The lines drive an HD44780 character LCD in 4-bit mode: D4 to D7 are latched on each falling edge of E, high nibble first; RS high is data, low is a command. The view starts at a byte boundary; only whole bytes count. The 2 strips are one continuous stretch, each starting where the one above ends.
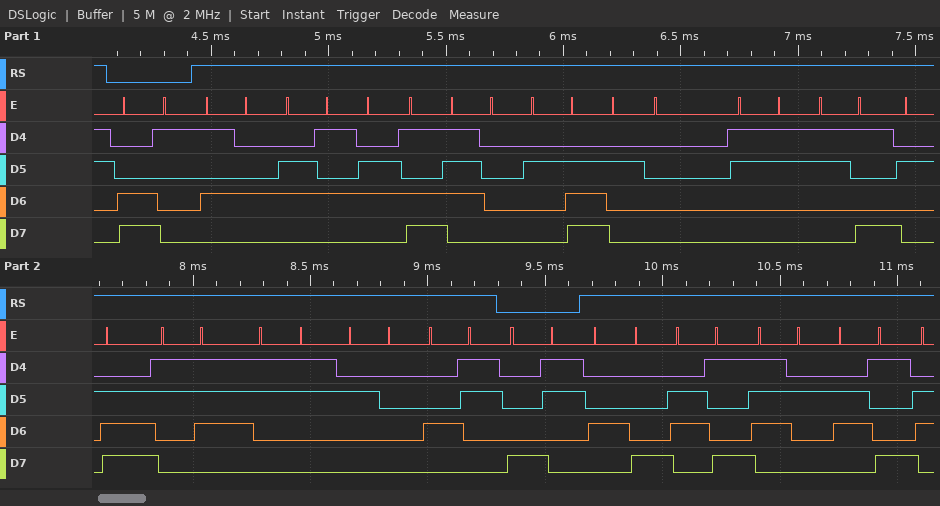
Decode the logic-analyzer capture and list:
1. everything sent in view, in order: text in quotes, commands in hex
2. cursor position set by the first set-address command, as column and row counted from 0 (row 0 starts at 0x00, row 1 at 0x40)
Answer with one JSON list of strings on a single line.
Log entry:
["0xC1 \"Temp. 39.73 C\" 0x83 \"Hiri\"", "column 1, row 1"]
